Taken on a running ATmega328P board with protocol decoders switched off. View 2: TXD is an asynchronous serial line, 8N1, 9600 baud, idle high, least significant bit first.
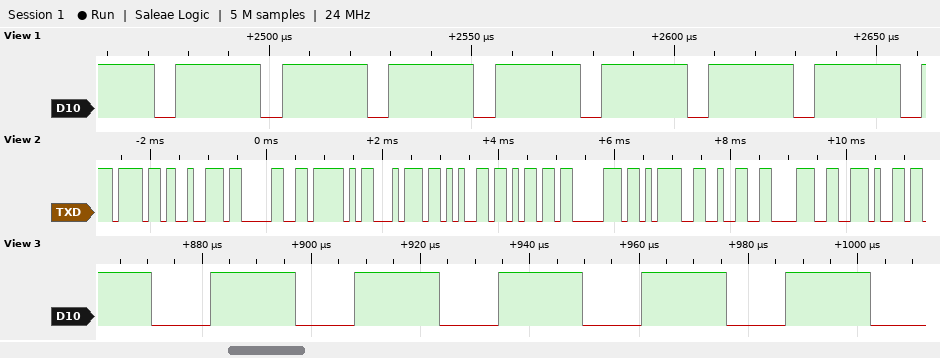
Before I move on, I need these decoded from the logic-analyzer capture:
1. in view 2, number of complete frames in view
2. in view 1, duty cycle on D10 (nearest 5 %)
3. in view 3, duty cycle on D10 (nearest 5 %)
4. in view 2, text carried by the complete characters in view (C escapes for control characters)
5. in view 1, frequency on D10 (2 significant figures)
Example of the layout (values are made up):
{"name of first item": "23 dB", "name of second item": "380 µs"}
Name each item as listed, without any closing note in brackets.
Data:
{"in view 2, number of complete frames in view": "12", "in view 1, duty cycle on D10": "80 %", "in view 3, duty cycle on D10": "60 %", "in view 2, text carried by the complete characters in view": "\"or0_temp=28.\"", "in view 1, frequency on D10": "38 kHz"}
